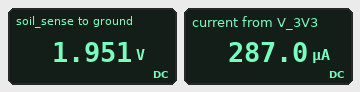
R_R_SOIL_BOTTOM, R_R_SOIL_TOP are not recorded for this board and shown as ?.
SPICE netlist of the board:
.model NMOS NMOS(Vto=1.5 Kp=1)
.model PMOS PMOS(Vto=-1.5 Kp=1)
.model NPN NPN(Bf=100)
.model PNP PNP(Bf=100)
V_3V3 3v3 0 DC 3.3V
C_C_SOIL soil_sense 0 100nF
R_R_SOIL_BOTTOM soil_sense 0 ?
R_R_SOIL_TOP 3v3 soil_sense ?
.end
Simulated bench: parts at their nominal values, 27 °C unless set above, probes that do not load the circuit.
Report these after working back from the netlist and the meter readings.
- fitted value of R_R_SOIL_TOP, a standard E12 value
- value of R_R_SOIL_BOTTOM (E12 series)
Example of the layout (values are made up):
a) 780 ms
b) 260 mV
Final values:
a) 4.7 kΩ
b) 6.8 kΩ
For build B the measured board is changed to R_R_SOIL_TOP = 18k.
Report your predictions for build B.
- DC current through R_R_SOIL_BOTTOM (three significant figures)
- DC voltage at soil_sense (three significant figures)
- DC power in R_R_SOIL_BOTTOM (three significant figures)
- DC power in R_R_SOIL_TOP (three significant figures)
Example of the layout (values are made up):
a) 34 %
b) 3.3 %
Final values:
a) 133 µA
b) 905 mV
c) 120 µW
d) 319 µW
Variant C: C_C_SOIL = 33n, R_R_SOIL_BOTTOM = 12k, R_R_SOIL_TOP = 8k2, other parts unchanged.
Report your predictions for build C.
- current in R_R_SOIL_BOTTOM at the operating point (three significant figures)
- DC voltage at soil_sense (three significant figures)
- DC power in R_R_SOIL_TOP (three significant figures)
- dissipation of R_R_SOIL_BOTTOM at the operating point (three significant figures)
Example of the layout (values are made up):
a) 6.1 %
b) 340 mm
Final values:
a) 163 µA
b) 1.96 V
c) 219 µW
d) 320 µW
